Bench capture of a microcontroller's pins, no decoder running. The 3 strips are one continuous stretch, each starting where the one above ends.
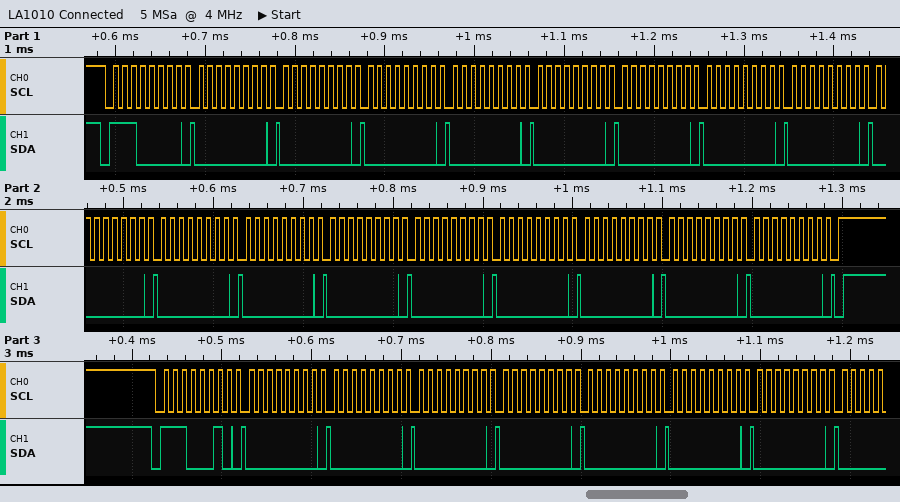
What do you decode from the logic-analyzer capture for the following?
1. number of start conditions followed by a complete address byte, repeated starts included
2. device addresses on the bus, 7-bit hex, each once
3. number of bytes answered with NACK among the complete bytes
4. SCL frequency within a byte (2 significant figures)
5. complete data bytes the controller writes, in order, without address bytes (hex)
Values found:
2
0x70 0x71
0
100 kHz
00 00 00 00 00 00 00 00 00 00 00 00 00 00 00 00 00 00 00 00 00 00 00 00
